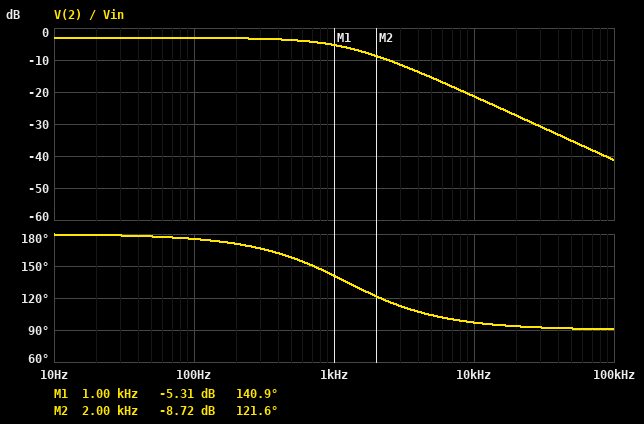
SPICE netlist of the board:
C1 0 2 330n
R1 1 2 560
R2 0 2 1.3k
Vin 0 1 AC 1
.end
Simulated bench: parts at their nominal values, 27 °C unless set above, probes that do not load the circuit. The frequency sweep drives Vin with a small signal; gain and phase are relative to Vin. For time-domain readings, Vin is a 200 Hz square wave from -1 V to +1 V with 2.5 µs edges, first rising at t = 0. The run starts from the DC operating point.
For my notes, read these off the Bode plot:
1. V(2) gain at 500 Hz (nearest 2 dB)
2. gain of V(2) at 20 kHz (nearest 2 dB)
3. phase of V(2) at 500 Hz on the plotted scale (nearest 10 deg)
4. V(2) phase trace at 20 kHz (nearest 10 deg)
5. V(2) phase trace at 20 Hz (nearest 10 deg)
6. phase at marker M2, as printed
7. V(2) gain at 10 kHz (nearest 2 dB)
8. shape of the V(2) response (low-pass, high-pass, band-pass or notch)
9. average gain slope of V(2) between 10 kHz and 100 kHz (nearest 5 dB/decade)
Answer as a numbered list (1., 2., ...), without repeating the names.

1. -4 dB
2. -28 dB
3. 160 deg
4. 90 deg
5. 180 deg
6. 121.6 deg
7. -22 dB
8. low-pass
9. -20 dB/decade
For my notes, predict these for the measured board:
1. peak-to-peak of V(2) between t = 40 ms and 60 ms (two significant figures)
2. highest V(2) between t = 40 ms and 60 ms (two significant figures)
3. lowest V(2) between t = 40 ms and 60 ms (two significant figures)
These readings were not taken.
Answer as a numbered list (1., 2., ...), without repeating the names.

1. 1.4 V
2. 700 mV
3. -700 mV
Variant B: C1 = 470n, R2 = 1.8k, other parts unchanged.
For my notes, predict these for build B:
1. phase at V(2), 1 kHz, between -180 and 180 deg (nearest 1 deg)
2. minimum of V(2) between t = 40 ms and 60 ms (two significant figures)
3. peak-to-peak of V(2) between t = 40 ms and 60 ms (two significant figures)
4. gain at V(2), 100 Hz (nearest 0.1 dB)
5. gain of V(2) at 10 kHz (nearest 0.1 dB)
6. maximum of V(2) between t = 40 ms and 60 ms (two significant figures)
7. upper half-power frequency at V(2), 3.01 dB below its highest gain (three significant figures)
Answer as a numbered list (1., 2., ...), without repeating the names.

1. 128 deg
2. -760 mV
3. 1.5 V
4. -2.4 dB
5. -24.4 dB
6. 760 mV
7. 793 Hz
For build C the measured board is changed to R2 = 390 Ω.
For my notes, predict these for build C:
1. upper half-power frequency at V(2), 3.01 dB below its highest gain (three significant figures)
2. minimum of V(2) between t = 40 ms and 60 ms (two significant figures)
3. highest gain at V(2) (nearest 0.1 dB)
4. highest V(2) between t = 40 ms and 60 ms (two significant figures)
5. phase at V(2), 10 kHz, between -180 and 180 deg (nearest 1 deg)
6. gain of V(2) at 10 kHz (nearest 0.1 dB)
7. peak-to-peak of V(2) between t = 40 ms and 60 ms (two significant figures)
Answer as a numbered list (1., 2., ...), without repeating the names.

1. 2.10 kHz
2. -410 mV
3. -7.7 dB
4. 410 mV
5. 102 deg
6. -21.5 dB
7. 820 mV
